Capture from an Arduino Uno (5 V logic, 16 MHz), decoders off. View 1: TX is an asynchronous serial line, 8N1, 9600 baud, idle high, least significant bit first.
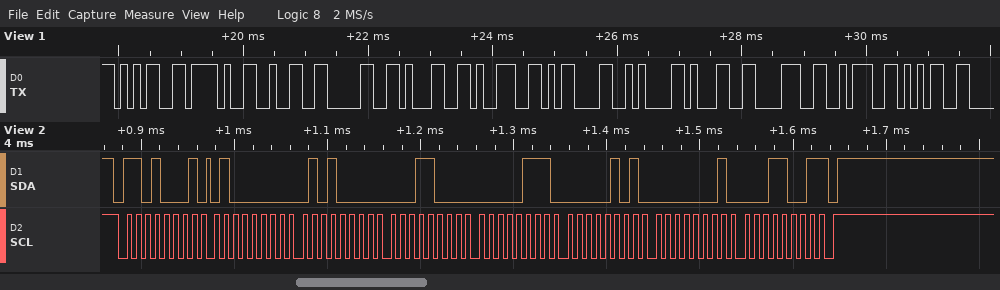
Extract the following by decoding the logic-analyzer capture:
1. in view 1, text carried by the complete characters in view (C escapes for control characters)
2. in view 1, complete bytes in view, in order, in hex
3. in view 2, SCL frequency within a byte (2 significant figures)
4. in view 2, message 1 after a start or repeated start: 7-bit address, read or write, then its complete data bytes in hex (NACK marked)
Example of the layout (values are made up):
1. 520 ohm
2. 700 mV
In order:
1. "5/2019\r\n18:5"
2. 0x35 0x2F 0x32 0x30 0x31 0x39 0x0D 0x0A 0x31 0x38 0x3A 0x35
3. 100 kHz
4. 0x68 read: 40 50 18 07 05 01 19 NACK
